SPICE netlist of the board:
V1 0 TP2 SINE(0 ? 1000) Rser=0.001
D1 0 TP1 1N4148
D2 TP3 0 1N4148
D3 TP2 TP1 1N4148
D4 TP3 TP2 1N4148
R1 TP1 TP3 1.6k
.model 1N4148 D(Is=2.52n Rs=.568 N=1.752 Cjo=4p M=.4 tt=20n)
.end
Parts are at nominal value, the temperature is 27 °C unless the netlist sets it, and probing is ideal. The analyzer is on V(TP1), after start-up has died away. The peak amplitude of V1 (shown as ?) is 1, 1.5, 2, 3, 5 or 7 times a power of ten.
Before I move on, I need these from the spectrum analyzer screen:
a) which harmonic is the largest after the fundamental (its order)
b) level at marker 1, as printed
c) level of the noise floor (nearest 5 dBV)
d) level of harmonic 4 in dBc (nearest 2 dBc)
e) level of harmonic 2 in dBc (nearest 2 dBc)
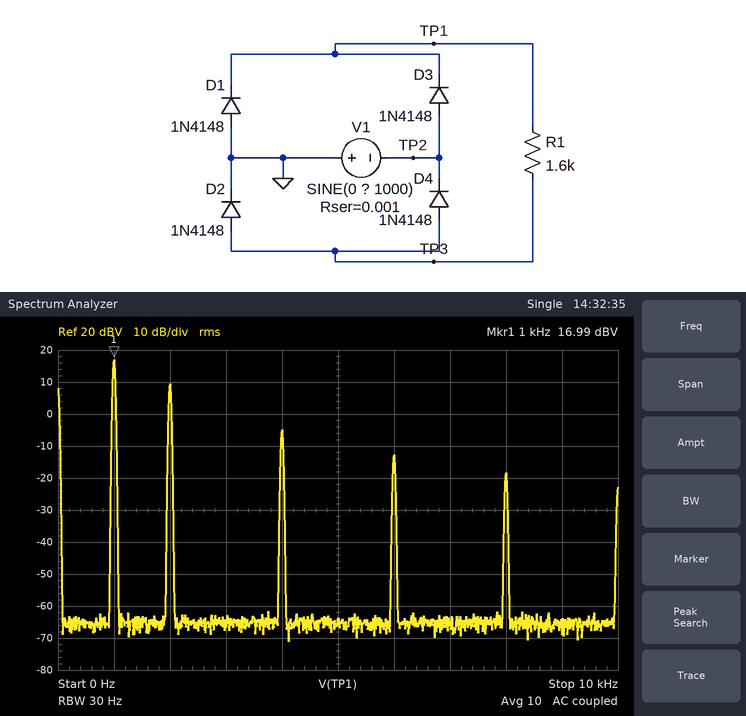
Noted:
2
16.99 dBV
-65 dBV
-22 dBc
-8 dBc
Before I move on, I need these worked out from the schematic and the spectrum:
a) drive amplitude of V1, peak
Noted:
20 V
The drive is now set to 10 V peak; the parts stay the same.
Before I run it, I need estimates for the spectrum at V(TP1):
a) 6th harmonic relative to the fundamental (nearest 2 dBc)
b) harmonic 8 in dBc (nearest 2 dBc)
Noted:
-32 dBc
-38 dBc
